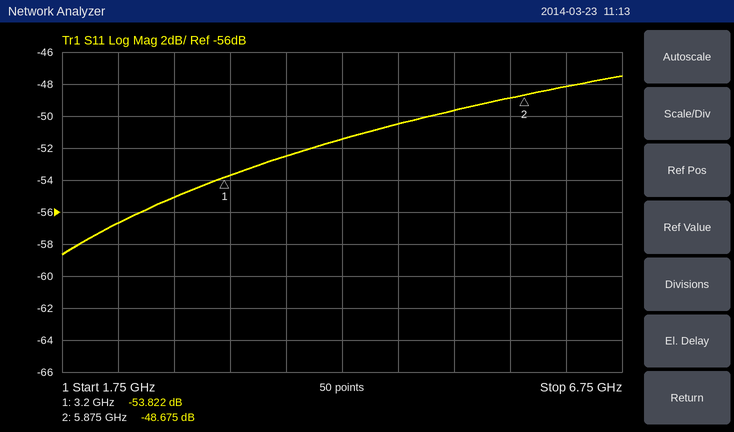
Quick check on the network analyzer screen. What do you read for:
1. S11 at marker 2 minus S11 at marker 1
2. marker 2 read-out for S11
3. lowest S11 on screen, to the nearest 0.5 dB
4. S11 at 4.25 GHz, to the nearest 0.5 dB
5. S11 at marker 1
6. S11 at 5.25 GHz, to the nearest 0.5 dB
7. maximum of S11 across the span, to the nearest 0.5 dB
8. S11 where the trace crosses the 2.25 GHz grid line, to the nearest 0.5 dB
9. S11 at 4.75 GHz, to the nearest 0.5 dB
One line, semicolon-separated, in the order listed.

5.147 dB; -48.675 dB; -58.5 dB; -51.5 dB; -53.822 dB; -49.5 dB; -47.5 dB; -56.5 dB; -50.5 dB
